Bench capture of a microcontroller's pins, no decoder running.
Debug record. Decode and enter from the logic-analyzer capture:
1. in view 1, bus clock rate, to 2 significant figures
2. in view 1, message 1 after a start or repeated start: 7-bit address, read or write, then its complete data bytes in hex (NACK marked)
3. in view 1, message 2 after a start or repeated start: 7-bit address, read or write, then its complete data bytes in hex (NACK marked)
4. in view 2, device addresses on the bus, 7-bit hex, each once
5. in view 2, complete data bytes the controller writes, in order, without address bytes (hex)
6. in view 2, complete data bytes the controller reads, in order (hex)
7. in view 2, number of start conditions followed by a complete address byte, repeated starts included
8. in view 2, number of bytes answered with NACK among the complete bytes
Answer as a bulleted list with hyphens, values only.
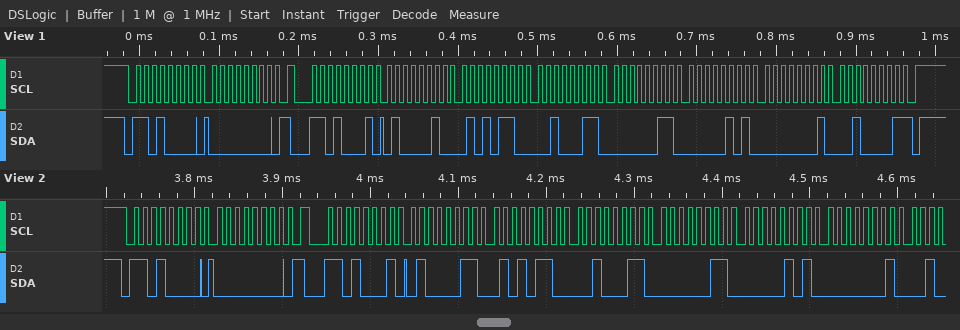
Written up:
- 100 kHz
- 0x68 write: 00
- 0x68 read: 42 56 23 03 05 01 21 NACK
- 0x68
- 00
- 43 56 23 03 05 01
- 2
- 0
